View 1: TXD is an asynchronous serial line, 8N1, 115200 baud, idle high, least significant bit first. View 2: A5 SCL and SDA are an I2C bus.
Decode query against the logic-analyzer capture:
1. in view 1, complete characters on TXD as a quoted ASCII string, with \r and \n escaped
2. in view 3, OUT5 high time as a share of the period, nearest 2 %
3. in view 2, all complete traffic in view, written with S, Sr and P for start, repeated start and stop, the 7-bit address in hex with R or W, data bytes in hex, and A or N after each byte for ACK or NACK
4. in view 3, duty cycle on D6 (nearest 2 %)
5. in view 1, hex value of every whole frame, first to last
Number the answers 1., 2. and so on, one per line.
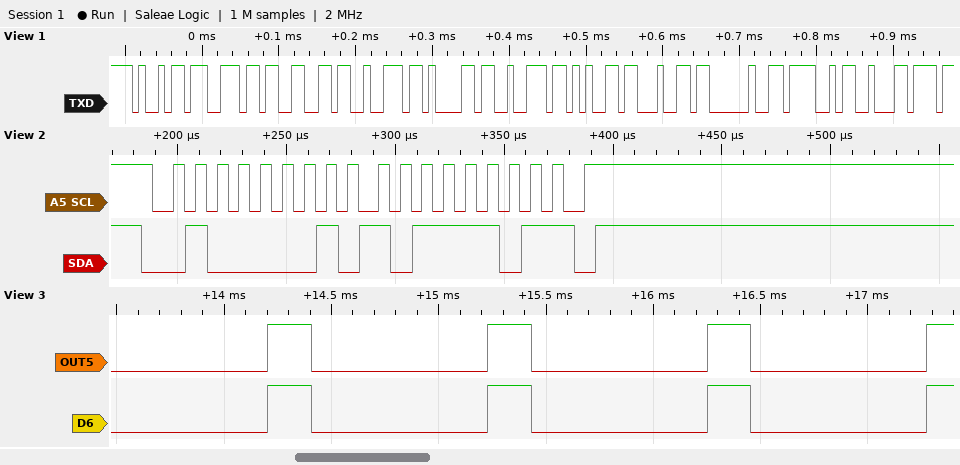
1. "infrared Ob"
2. 20 %
3. S 20R A BD N P
4. 20 %
5. 69 6E 66 72 61 72 65 64 20 4F 62
